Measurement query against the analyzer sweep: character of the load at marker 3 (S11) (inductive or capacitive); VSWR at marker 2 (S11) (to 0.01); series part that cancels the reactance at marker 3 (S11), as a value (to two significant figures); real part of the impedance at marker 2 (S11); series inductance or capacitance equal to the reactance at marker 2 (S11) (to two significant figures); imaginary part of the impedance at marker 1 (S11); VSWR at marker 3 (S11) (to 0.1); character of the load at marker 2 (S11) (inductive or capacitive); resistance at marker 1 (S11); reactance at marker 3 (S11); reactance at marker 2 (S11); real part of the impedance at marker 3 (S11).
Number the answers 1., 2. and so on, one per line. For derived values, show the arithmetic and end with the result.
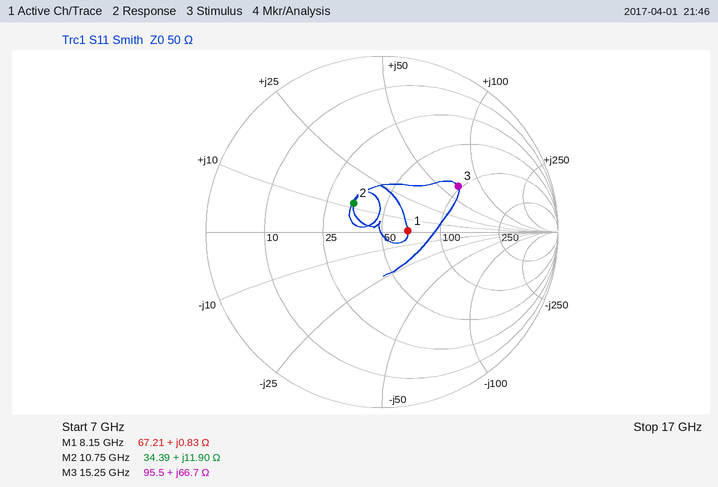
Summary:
1. inductive
2. 1.60
3. C = 1/(2π × 15.25 GHz × 66.7 Ω) ≈ 156 fF, so 160 fF to two significant figures
4. 34.39 Ω
5. L = 11.9 Ω/(2π × 10.75 GHz) ≈ 176 pH, so 180 pH to two significant figures
6. +0.83 Ω
7. 3.0
8. inductive
9. 67.21 Ω
10. +66.7 Ω
11. +11.90 Ω
12. 95.5 Ω
